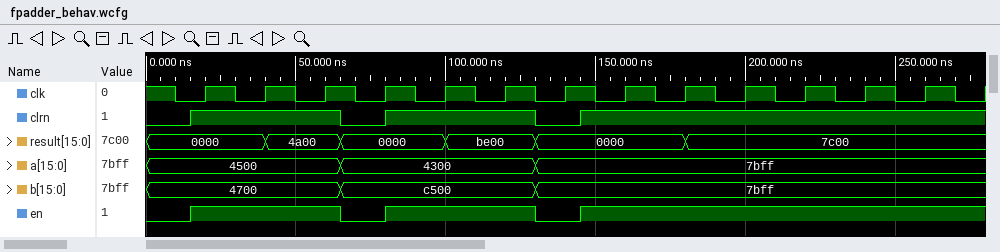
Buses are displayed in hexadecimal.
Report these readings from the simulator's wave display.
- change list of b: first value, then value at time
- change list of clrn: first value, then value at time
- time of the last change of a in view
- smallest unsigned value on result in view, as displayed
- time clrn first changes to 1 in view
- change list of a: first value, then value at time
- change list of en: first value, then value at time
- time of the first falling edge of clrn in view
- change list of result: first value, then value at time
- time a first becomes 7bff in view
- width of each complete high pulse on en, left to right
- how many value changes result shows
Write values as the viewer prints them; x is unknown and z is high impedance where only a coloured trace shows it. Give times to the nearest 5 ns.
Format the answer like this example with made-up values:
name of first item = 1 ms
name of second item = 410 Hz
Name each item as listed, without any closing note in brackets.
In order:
change list of b: first value, then value at time = 4700, c500 at 65 ns, 7bff at 130 ns
change list of clrn: first value, then value at time = 0, 1 at 15 ns, 0 at 65 ns, 1 at 80 ns, 0 at 130 ns, 1 at 145 ns
time of the last change of a in view = 130 ns
smallest unsigned value on result in view, as displayed = 0000
time clrn first changes to 1 in view = 15 ns
change list of a: first value, then value at time = 4500, 4300 at 65 ns, 7bff at 130 ns
change list of en: first value, then value at time = 0, 1 at 15 ns, 0 at 65 ns, 1 at 80 ns, 0 at 130 ns, 1 at 145 ns
time of the first falling edge of clrn in view = 65 ns
change list of result: first value, then value at time = 0000, 4a00 at 40 ns, 0000 at 65 ns, be00 at 100 ns, 0000 at 130 ns, 7c00 at 180 ns
time a first becomes 7bff in view = 130 ns
width of each complete high pulse on en, left to right = 50 ns, 50 ns
how many value changes result shows = 5
